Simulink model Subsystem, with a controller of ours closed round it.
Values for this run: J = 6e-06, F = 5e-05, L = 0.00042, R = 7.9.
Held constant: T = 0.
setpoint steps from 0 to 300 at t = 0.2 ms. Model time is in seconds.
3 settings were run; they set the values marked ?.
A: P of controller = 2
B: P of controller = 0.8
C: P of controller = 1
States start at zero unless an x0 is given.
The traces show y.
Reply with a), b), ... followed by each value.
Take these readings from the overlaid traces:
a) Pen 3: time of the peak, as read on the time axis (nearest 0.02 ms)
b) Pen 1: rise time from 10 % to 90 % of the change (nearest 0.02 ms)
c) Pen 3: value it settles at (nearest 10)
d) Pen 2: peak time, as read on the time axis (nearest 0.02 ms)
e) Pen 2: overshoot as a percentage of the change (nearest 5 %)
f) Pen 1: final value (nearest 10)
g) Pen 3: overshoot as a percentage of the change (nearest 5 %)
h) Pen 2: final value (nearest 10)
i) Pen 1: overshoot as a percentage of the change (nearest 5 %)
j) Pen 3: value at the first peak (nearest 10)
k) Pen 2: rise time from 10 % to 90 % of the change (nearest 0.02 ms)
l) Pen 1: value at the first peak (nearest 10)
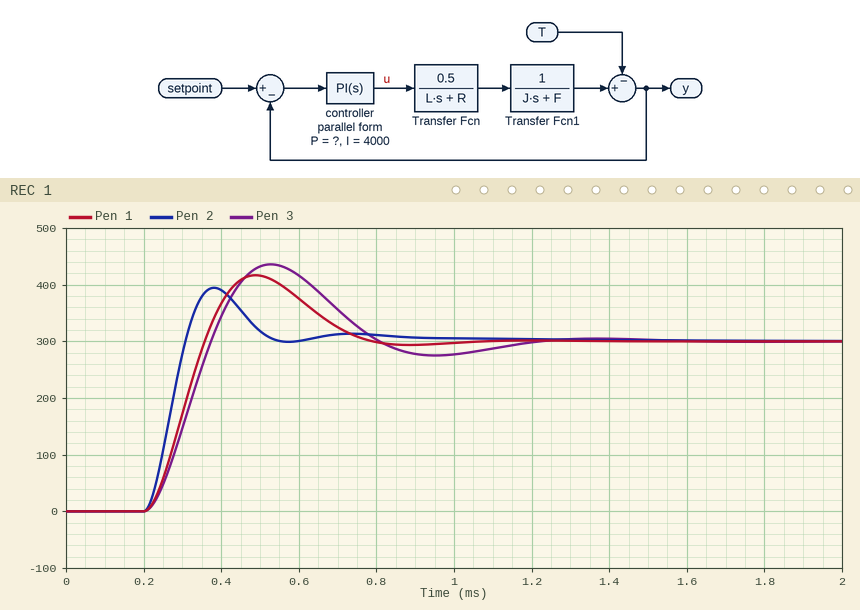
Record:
a) 0.52 ms
b) 0.10 ms
c) 300
d) 0.38 ms
e) 30 %
f) 300
g) 45 %
h) 300
i) 40 %
j) 440
k) 0.08 ms
l) 420
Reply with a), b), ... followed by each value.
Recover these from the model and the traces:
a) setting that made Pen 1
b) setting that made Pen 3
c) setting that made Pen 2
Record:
a) C
b) B
c) A
